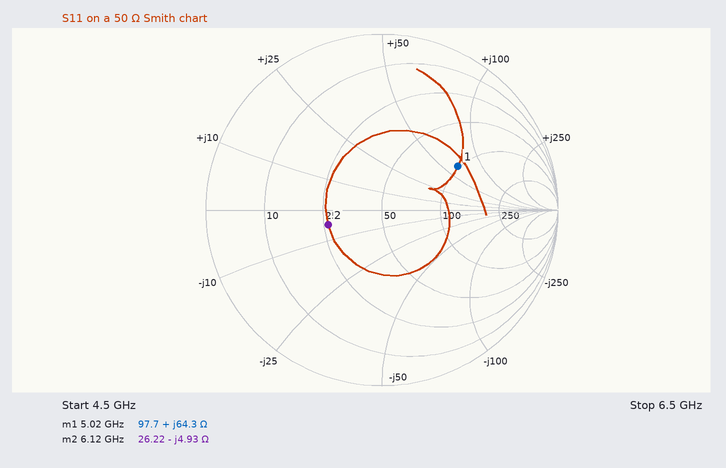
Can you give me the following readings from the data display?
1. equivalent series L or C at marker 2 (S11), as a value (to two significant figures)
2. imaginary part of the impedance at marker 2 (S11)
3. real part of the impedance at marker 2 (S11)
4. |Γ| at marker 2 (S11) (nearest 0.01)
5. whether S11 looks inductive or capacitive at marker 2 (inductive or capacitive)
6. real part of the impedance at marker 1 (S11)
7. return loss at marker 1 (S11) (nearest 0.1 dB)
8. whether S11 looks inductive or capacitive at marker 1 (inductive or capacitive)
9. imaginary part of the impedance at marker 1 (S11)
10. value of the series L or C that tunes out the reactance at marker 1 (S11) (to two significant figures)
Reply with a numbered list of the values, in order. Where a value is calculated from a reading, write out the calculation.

1. C = 1/(2π × 6.12 GHz × 4.93 Ω) ≈ 5.3 pF
2. -4.93 Ω
3. 26.22 Ω
4. 0.32
5. capacitive
6. 97.7 Ω
7. 6.1 dB
8. inductive
9. +64.3 Ω
10. C = 1/(2π × 5.02 GHz × 64.3 Ω) ≈ 493 fF, so 490 fF to two significant figures
